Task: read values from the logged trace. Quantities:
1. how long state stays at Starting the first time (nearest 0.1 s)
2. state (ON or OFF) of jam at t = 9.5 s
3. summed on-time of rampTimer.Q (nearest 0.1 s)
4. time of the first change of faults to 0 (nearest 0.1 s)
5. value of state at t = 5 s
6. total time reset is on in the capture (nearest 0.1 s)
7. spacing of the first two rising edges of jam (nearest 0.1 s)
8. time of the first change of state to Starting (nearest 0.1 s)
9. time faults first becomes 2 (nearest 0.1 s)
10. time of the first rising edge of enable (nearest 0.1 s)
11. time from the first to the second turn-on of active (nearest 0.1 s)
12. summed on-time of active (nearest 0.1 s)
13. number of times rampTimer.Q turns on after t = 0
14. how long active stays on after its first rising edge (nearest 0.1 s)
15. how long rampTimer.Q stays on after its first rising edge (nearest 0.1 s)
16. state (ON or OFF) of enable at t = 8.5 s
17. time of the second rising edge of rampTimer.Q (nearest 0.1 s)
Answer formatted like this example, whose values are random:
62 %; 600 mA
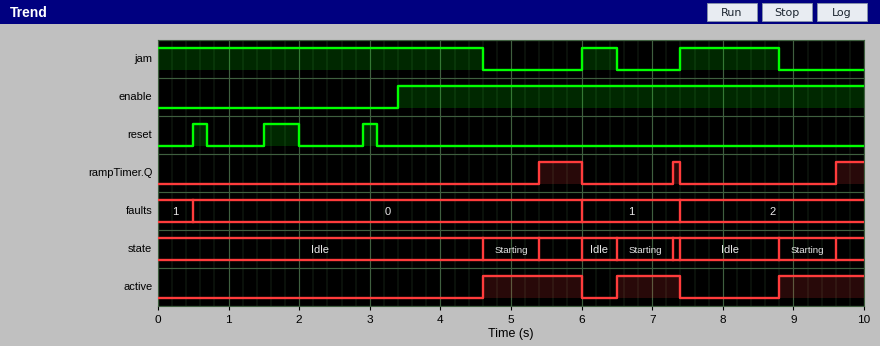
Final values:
0.8 s; OFF; 1.1 s; 0.5 s; Starting; 0.9 s; 1.4 s; 4.6 s; 7.4 s; 3.4 s; 1.9 s; 3.5 s; 3; 1.4 s; 0.6 s; ON; 7.3 s
